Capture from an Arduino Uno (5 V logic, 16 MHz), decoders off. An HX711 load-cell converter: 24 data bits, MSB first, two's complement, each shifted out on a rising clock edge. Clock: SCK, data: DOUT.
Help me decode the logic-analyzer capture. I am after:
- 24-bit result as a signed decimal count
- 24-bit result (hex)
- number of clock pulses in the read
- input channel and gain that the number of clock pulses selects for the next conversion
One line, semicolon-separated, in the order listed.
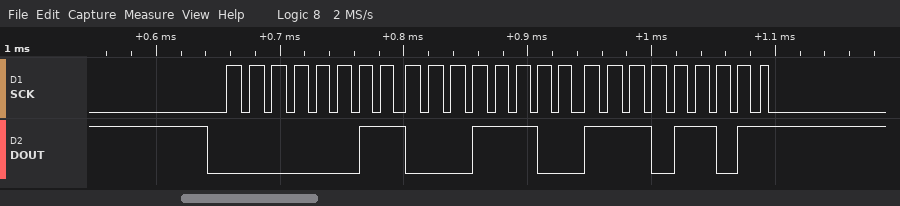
204013; 0x031CED; 25; channel A, gain 128
